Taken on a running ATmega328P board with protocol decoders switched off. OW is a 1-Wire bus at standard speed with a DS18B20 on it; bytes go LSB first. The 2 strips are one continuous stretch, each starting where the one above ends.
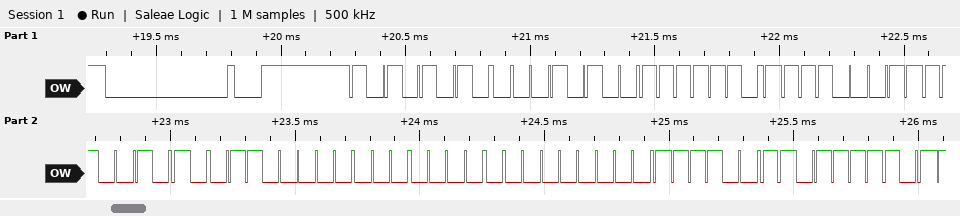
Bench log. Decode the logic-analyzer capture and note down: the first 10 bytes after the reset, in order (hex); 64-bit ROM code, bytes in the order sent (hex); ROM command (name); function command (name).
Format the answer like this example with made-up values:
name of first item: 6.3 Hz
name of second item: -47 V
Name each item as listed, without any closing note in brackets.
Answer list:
the first 10 bytes after the reset, in order: 55 28 BF C7 53 06 00 00 CF BE
64-bit ROM code, bytes in the order sent: 28 BF C7 53 06 00 00 CF
ROM command: Match ROM
function command: Read Scratchpad
